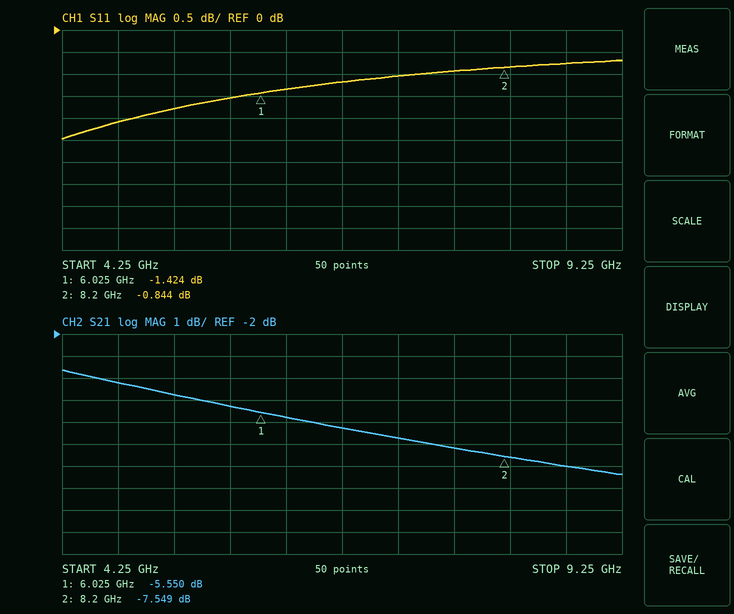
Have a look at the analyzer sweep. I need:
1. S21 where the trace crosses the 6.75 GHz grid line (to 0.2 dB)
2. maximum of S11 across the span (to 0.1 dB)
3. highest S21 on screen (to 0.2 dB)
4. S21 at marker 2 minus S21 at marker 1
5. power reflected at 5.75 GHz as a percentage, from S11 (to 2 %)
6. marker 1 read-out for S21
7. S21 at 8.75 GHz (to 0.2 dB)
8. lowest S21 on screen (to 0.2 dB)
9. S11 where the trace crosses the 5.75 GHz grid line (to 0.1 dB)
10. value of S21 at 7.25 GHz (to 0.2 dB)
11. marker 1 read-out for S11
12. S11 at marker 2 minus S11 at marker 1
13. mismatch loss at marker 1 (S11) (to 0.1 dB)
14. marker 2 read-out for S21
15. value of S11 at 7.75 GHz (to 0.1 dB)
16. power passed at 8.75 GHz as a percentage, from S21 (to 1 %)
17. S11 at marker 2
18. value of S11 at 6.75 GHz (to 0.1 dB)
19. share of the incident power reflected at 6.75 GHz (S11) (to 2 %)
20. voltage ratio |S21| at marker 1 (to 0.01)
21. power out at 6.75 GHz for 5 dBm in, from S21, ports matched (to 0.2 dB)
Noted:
-6.2 dB
-0.7 dB
-3.6 dB
-1.999 dB
70 %
-5.550 dB
-8.0 dB
-8.4 dB
-1.5 dB
-6.8 dB
-1.424 dB
0.580 dB
5.5 dB
-7.549 dB
-0.9 dB
16 %
-0.844 dB
-1.2 dB
76 %
0.53
-1.2 dBm
